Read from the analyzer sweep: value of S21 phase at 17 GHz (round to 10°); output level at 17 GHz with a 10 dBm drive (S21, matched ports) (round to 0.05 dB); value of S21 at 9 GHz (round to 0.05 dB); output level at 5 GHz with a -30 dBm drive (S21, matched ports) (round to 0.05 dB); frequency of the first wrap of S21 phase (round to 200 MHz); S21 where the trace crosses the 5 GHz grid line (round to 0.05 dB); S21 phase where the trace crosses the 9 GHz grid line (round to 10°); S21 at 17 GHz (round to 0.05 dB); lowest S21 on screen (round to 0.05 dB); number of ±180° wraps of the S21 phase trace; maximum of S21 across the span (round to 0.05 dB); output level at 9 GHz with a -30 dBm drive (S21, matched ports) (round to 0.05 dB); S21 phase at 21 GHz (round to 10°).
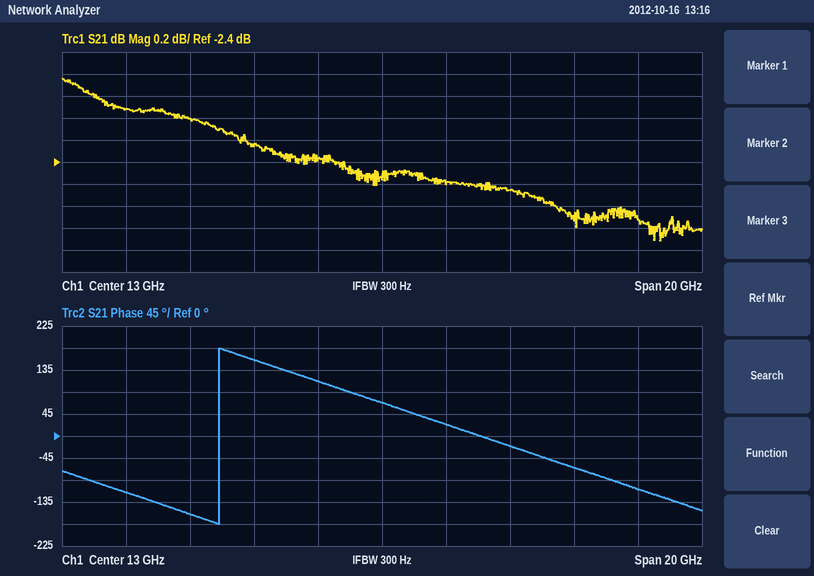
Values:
-20°
7.35 dBm
-2.25 dB
-31.90 dBm
8.0 GHz
-1.90 dB
160°
-2.65 dB
-3.10 dB
1
-1.65 dB
-32.25 dBm
-110°
